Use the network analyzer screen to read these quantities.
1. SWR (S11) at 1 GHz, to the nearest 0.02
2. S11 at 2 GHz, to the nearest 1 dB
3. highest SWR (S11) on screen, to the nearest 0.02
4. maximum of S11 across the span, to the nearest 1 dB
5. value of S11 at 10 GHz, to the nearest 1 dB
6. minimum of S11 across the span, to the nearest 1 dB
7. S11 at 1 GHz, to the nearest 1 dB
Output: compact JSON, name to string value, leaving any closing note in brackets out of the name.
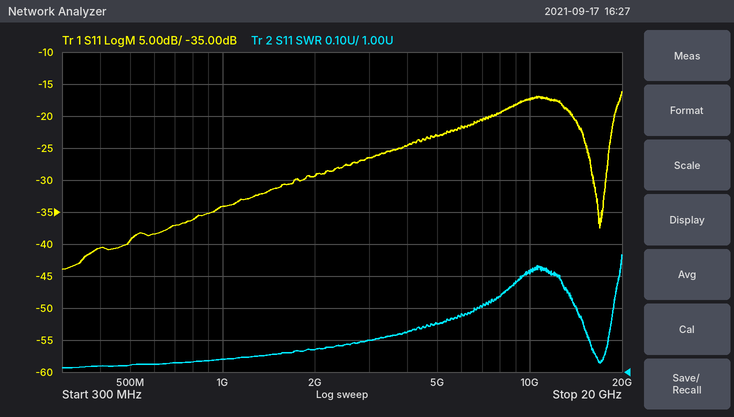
{"SWR (S11) at 1 GHz, to the nearest 0.02": "1.04", "S11 at 2 GHz, to the nearest 1 dB": "-29 dB", "highest SWR (S11) on screen, to the nearest 0.02": "1.36", "maximum of S11 across the span, to the nearest 1 dB": "-16 dB", "value of S11 at 10 GHz, to the nearest 1 dB": "-17 dB", "minimum of S11 across the span, to the nearest 1 dB": "-44 dB", "S11 at 1 GHz, to the nearest 1 dB": "-34 dB"}
